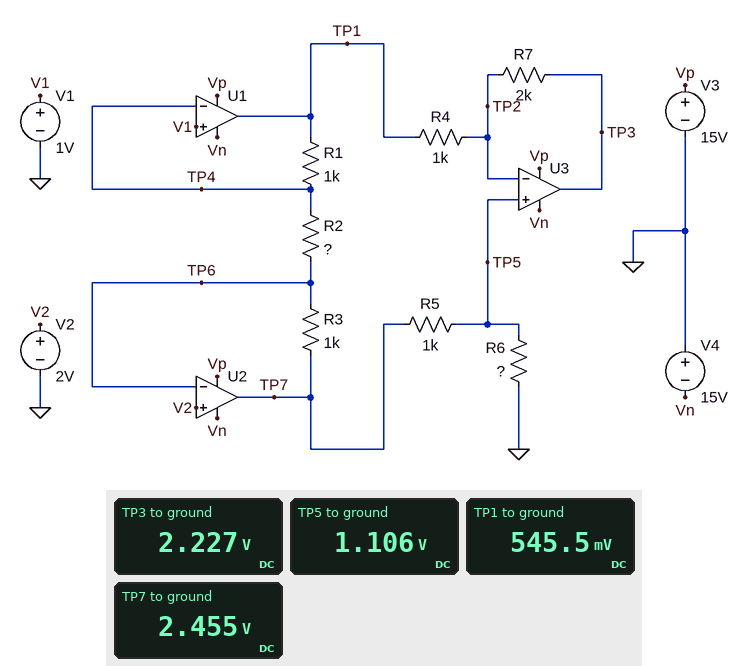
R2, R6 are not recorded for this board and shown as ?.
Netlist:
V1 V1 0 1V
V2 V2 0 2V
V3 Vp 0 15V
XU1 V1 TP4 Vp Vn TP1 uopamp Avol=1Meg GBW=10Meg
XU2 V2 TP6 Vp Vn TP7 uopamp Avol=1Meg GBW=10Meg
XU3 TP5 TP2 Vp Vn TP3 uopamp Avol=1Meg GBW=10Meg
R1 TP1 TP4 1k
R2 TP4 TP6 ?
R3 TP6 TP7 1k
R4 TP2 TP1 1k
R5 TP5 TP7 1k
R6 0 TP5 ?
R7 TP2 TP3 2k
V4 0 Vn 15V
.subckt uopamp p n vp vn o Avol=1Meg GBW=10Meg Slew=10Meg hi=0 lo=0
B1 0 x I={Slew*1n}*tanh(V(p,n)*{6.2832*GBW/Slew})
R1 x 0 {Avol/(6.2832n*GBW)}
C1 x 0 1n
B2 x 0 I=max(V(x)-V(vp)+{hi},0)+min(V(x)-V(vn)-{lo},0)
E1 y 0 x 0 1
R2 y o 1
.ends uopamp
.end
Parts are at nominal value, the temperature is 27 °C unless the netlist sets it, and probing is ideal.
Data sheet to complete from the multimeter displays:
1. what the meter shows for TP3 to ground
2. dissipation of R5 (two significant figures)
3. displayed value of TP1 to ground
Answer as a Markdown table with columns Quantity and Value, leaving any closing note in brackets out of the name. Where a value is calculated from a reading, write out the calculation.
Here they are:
| Quantity | Value |
|---|---|
| what the meter shows for TP3 to ground | 2.227 V |
| dissipation of R5 | (2.455 V - 1.106 V)^2 / 1 kΩ = 1.8 mW |
| displayed value of TP1 to ground | 545.5 mV |
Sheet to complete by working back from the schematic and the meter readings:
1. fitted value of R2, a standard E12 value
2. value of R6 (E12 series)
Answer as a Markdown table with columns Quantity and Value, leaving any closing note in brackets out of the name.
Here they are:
| Quantity | Value |
|---|---|
| fitted value of R2, a standard E12 value | 2.2 kΩ |
| value of R6 | 820 Ω |
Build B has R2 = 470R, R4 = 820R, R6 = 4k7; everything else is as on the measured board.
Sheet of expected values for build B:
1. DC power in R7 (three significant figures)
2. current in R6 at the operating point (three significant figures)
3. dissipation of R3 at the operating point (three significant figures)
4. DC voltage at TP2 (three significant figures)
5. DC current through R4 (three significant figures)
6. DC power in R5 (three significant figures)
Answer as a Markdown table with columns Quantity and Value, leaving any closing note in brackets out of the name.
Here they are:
| Quantity | Value |
|---|---|
| DC power in R7 | 61.1 mW |
| current in R6 at the operating point | 724 µA |
| dissipation of R3 at the operating point | 4.53 mW |
| DC voltage at TP2 | 3.40 V |
| DC current through R4 | 5.53 mA |
| DC power in R5 | 524 µW |
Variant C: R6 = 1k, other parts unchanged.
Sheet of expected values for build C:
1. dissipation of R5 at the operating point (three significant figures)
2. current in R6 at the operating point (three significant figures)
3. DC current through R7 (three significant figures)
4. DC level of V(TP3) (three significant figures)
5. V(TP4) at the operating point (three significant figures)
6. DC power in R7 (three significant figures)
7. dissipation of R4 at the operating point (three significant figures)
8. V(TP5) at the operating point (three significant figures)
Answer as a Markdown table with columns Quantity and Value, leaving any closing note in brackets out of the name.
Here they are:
| Quantity | Value |
|---|---|
| dissipation of R5 at the operating point | 1.51 mW |
| current in R6 at the operating point | 1.23 mA |
| DC current through R7 | 682 µA |
| DC level of V(TP3) | 2.59 V |
| V(TP4) at the operating point | 1.00 V |
| DC power in R7 | 930 µW |
| dissipation of R4 at the operating point | 465 µW |
| V(TP5) at the operating point | 1.23 V |
